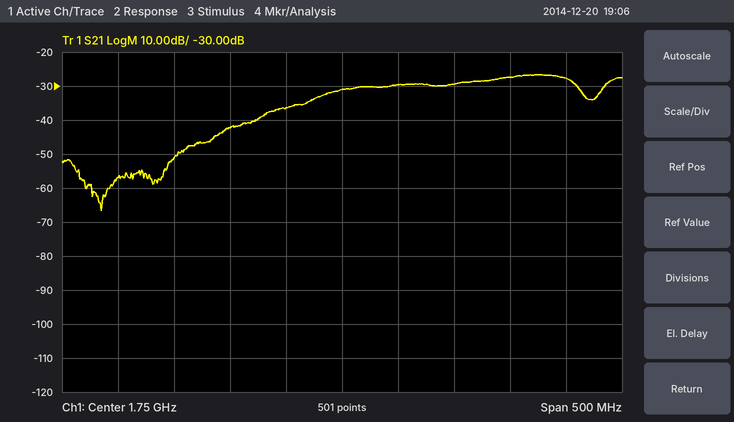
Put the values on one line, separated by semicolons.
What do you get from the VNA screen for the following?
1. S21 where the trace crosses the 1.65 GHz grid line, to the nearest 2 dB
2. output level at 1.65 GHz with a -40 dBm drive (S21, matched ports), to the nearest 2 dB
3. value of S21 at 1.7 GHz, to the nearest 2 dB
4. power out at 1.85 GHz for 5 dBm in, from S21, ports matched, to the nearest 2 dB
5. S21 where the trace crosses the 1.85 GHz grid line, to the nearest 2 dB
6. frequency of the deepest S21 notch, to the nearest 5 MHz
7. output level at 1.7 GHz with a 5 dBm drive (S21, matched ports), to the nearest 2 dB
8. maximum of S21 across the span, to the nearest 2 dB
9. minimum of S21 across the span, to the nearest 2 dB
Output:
-42 dB; -82 dBm; -36 dB; -24 dBm; -30 dB; 1.535 GHz; -32 dBm; -26 dB; -66 dB
